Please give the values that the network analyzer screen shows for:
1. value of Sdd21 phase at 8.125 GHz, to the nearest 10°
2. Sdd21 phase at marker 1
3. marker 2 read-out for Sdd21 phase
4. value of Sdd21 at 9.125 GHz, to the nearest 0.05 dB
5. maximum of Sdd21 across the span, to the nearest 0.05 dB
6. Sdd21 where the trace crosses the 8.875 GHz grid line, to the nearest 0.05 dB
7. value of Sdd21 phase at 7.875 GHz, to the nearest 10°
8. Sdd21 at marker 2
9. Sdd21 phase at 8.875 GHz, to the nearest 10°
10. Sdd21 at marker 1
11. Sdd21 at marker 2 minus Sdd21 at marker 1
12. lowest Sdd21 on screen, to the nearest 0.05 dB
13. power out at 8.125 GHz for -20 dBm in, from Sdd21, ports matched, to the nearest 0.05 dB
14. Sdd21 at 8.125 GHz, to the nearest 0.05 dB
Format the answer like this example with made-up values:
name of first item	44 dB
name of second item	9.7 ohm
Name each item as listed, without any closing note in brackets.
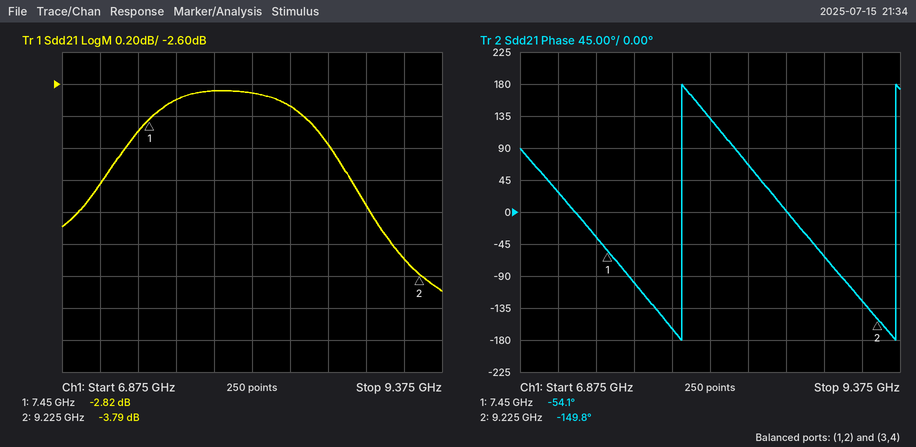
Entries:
value of Sdd21 phase at 8.125 GHz, to the nearest 10°	130°
Sdd21 phase at marker 1	-54.1°
marker 2 read-out for Sdd21 phase	-149.8°
value of Sdd21 at 9.125 GHz, to the nearest 0.05 dB	-3.70 dB
maximum of Sdd21 across the span, to the nearest 0.05 dB	-2.65 dB
Sdd21 where the trace crosses the 8.875 GHz grid line, to the nearest 0.05 dB	-3.35 dB
value of Sdd21 phase at 7.875 GHz, to the nearest 10°	-160°
Sdd21 at marker 2	-3.79 dB
Sdd21 phase at 8.875 GHz, to the nearest 10°	-60°
Sdd21 at marker 1	-2.82 dB
Sdd21 at marker 2 minus Sdd21 at marker 1	-0.97 dB
lowest Sdd21 on screen, to the nearest 0.05 dB	-3.90 dB
power out at 8.125 GHz for -20 dBm in, from Sdd21, ports matched, to the nearest 0.05 dB	-22.65 dBm
Sdd21 at 8.125 GHz, to the nearest 0.05 dB	-2.65 dB
